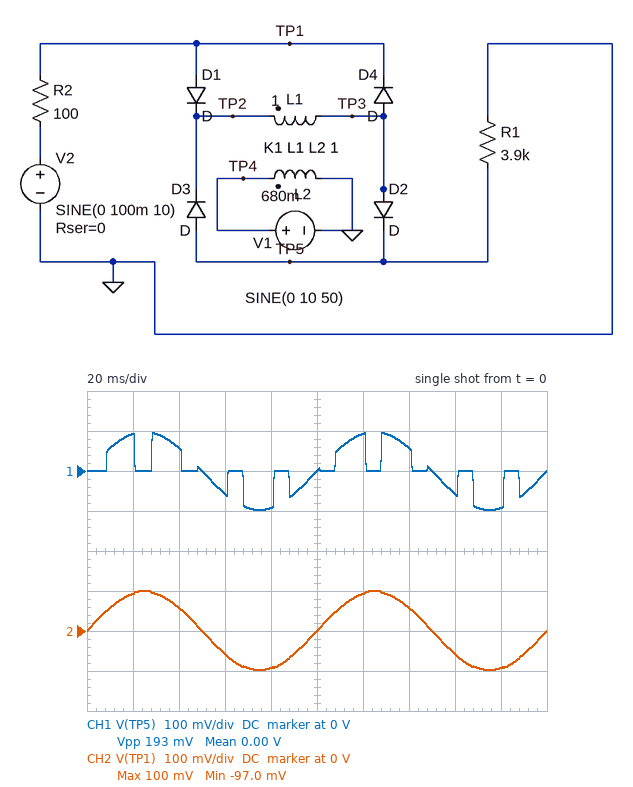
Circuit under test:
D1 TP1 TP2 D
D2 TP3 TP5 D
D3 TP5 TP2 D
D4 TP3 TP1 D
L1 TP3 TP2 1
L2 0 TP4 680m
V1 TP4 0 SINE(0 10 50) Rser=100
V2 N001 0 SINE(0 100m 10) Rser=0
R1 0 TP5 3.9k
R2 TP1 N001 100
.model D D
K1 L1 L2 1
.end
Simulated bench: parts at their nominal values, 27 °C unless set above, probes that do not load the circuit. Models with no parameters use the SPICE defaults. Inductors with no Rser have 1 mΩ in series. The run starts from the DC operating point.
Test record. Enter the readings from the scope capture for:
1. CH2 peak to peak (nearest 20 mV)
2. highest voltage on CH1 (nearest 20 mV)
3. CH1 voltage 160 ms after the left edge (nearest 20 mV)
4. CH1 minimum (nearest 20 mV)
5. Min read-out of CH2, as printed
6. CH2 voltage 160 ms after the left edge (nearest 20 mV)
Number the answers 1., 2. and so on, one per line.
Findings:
1. 200 mV
2. 100 mV
3. -60 mV
4. -100 mV
5. -97.0 mV
6. -60 mV
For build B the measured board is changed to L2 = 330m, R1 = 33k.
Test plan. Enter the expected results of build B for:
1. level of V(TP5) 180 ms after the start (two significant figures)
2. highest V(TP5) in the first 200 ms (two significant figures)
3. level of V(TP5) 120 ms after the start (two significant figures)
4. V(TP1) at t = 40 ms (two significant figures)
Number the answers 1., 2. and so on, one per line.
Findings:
1. -95 mV
2. 98 mV
3. 95 mV
4. 59 mV
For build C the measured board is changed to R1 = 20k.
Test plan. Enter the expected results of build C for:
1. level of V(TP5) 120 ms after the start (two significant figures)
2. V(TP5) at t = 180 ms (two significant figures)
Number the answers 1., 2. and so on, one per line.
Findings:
1. 95 mV
2. -95 mV
